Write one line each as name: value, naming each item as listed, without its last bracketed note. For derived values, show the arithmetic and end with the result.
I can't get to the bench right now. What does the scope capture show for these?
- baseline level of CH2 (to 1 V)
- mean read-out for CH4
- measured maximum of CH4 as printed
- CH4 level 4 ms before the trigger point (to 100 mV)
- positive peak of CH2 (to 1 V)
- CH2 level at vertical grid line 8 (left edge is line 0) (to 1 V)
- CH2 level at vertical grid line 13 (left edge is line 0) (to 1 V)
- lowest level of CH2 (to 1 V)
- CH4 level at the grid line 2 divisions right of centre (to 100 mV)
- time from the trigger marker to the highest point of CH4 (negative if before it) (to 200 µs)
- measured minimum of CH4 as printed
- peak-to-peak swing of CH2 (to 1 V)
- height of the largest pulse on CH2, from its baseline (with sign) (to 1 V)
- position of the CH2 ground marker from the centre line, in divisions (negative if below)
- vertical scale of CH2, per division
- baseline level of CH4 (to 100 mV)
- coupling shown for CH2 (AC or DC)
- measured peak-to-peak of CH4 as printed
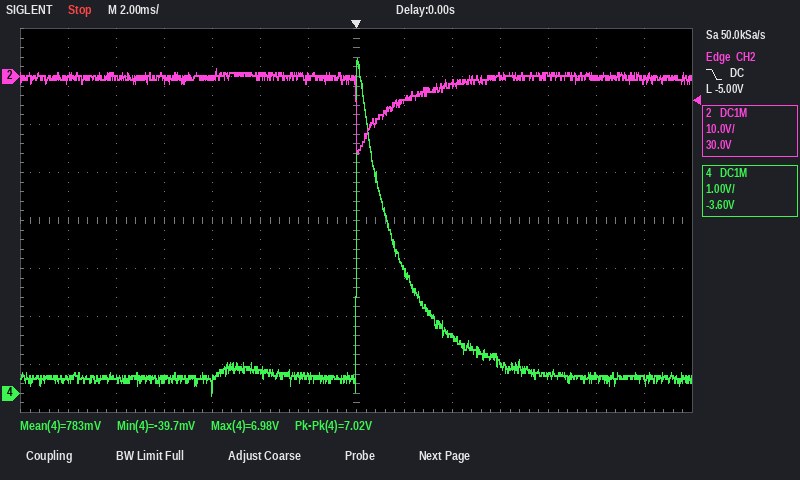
baseline level of CH2: 0 V
mean read-out for CH4: 783 mV
measured maximum of CH4 as printed: 6.98 V
CH4 level 4 ms before the trigger point: 500 mV
positive peak of CH2: 2 V
CH2 level at vertical grid line 8 (left edge is line 0): -5 V
CH2 level at vertical grid line 13 (left edge is line 0): -1 V
lowest level of CH2: -16 V
CH4 level at the grid line 2 divisions right of centre: 1.2 V
time from the trigger marker to the highest point of CH4 (negative if before it): 0.0 ms
measured minimum of CH4 as printed: -39.7 mV
peak-to-peak swing of CH2: 2 V − (-16 V) = 18 V
height of the largest pulse on CH2, from its baseline (with sign): -16 V − (0 V) = -16 V
position of the CH2 ground marker from the centre line, in divisions: +3.0 div
vertical scale of CH2, per division: 10 V
baseline level of CH4: 300 mV
coupling shown for CH2: DC
measured peak-to-peak of CH4 as printed: 7.02 V
